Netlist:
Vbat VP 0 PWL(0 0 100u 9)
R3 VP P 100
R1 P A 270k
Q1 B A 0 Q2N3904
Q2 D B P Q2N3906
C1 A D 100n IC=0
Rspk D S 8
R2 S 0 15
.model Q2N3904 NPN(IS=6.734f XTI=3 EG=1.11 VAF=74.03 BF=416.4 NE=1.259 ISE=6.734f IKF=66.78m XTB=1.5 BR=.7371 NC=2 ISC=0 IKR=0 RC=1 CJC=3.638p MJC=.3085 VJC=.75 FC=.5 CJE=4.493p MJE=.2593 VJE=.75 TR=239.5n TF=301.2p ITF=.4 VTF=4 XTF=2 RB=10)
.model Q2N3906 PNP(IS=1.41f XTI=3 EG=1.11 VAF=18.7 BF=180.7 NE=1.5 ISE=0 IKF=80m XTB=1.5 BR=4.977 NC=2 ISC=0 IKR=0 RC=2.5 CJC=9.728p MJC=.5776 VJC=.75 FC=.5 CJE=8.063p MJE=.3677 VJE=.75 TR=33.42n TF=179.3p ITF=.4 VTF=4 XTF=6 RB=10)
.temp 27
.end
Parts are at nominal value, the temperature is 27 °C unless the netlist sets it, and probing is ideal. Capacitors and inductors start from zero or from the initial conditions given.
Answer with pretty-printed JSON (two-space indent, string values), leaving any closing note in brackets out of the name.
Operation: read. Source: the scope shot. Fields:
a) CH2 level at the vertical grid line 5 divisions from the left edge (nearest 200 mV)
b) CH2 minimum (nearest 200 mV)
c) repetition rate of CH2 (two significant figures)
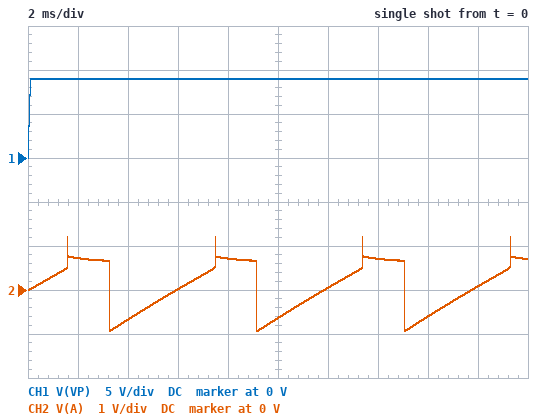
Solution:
{
  "CH2 level at the vertical grid line 5 divisions from the left edge": "-600 mV",
  "CH2 minimum": "-1.0 V",
  "repetition rate of CH2": "170 Hz"
}
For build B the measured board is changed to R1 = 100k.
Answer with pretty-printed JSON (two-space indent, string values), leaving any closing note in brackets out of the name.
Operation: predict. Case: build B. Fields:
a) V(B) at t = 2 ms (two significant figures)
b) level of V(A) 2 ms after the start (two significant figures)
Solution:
{
  "V(B) at t = 2 ms": "990 mV",
  "level of V(A) 2 ms after the start": "690 mV"
}
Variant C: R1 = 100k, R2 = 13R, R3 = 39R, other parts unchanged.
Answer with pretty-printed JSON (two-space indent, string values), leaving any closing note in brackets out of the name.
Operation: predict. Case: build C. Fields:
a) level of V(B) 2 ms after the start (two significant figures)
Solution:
{
  "level of V(B) 2 ms after the start": "2.5 V"
}
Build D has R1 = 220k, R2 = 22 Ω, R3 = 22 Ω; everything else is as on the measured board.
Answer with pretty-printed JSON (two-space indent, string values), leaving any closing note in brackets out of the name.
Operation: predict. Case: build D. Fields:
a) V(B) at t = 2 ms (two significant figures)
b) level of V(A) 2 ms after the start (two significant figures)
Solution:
{
  "V(B) at t = 2 ms": "4.4 V",
  "level of V(A) 2 ms after the start": "720 mV"
}
